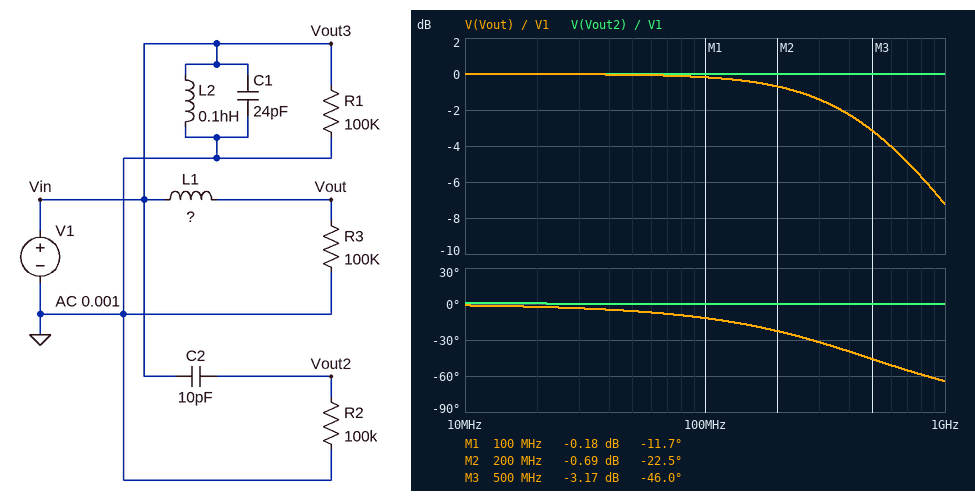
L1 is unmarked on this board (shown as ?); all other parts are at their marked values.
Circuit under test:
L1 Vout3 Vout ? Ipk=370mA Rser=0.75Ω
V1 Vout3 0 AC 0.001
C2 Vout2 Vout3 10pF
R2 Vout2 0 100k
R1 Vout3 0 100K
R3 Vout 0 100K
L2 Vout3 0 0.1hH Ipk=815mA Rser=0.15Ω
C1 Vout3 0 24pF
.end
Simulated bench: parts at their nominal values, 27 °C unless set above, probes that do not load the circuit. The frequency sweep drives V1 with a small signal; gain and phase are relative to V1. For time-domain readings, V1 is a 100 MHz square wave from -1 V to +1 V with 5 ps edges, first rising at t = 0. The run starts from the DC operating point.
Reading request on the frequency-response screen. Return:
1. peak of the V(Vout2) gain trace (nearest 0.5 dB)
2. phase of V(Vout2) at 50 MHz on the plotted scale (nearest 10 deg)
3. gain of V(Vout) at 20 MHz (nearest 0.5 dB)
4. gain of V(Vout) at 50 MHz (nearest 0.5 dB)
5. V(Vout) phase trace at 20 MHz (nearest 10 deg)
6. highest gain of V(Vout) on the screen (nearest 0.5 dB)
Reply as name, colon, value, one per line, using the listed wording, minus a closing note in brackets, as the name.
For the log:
peak of the V(Vout2) gain trace: 0 dB
phase of V(Vout2) at 50 MHz on the plotted scale: 0 deg
gain of V(Vout) at 20 MHz: 0 dB
gain of V(Vout) at 50 MHz: 0 dB
V(Vout) phase trace at 20 MHz: 0 deg
highest gain of V(Vout) on the screen: 0 dB
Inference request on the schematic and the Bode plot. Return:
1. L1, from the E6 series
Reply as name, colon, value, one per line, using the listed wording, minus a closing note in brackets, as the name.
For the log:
L1, from the E6 series: 33 µH
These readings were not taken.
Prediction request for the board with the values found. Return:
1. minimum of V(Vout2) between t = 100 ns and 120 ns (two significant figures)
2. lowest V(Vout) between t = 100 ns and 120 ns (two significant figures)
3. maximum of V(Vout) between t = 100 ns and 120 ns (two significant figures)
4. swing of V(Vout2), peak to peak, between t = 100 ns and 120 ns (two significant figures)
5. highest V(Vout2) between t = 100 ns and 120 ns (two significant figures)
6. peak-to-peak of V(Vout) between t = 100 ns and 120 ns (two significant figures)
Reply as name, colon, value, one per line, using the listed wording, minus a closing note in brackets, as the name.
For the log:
minimum of V(Vout2) between t = 100 ns and 120 ns: -110 mV
lowest V(Vout) between t = 100 ns and 120 ns: -1.0 V
maximum of V(Vout) between t = 100 ns and 120 ns: 1.0 V
swing of V(Vout2), peak to peak, between t = 100 ns and 120 ns: 2.0 V
highest V(Vout2) between t = 100 ns and 120 ns: 1.9 V
peak-to-peak of V(Vout) between t = 100 ns and 120 ns: 2.0 V
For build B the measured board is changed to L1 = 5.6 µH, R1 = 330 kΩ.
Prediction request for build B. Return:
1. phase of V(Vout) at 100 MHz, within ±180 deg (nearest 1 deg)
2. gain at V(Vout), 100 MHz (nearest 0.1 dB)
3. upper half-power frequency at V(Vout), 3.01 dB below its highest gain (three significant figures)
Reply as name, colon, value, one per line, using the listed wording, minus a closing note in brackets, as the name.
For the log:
phase of V(Vout) at 100 MHz, within ±180 deg: -2 deg
gain at V(Vout), 100 MHz: 0 dB
upper half-power frequency at V(Vout), 3.01 dB below its highest gain: 2.84 GHz
